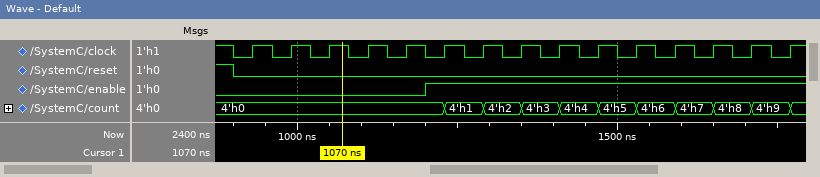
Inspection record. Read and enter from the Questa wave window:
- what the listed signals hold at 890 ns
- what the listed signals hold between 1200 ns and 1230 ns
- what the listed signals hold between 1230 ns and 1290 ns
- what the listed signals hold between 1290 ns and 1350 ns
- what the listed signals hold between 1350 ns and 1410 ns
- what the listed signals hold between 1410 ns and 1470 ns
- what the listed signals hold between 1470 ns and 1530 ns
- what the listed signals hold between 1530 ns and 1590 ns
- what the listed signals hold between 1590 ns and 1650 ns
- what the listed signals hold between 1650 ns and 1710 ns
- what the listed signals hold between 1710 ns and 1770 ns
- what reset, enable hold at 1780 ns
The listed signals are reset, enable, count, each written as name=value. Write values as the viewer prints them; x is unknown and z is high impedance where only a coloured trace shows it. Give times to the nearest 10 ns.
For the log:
reset=1, enable=0, count=4'h0
reset=0, enable=1, count=4'h0
reset=0, enable=1, count=4'h1
reset=0, enable=1, count=4'h2
reset=0, enable=1, count=4'h3
reset=0, enable=1, count=4'h4
reset=0, enable=1, count=4'h5
reset=0, enable=1, count=4'h6
reset=0, enable=1, count=4'h7
reset=0, enable=1, count=4'h8
reset=0, enable=1, count=4'h9
reset=0, enable=1
